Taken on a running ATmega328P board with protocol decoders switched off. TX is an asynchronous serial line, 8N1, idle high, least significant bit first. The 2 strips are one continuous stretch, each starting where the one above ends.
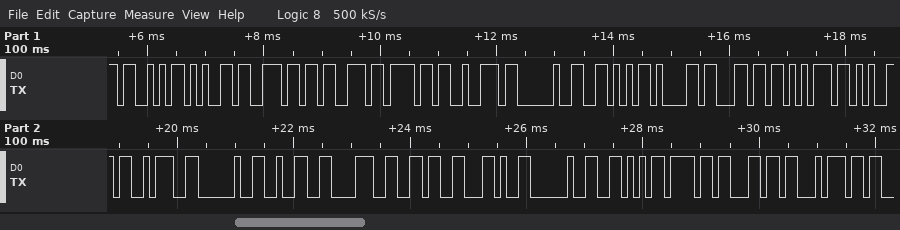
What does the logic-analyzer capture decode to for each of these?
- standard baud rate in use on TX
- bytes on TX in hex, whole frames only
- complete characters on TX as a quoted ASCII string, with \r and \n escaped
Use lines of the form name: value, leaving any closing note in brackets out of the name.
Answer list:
standard baud rate in use on TX: 9600 baud
bytes on TX in hex, whole frames only: 53 65 6E 73 6F 72 20 56 61 6C 75 65 3A 20 32 38 36 2C 20 56 6F 6C 74
complete characters on TX as a quoted ASCII string, with \r and \n escaped: "Sensor Value: 286, Volt"
